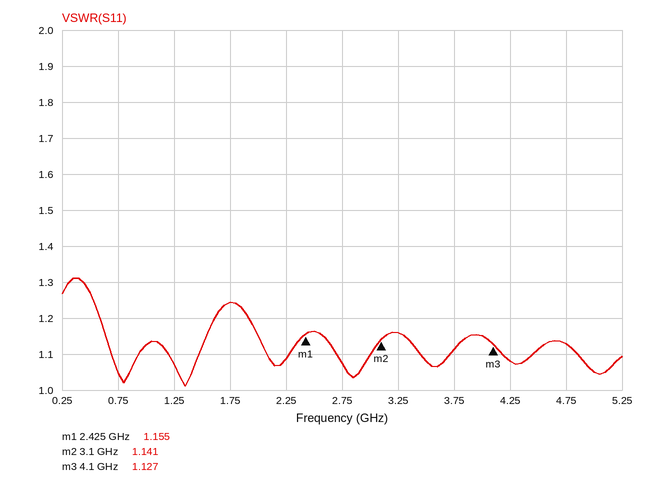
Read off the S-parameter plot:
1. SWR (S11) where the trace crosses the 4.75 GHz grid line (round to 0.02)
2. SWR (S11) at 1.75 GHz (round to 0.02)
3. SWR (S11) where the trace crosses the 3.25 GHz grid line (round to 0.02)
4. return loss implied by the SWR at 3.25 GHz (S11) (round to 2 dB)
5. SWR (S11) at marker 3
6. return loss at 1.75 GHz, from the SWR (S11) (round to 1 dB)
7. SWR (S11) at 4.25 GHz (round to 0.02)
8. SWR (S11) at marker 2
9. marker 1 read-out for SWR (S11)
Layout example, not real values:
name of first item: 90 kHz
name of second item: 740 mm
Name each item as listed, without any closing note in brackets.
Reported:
SWR (S11) where the trace crosses the 4.75 GHz grid line: 1.12
SWR (S11) at 1.75 GHz: 1.24
SWR (S11) where the trace crosses the 3.25 GHz grid line: 1.16
return loss implied by the SWR at 3.25 GHz (S11): 22 dB
SWR (S11) at marker 3: 1.127
return loss at 1.75 GHz, from the SWR (S11): 19 dB
SWR (S11) at 4.25 GHz: 1.08
SWR (S11) at marker 2: 1.141
marker 1 read-out for SWR: 1.155
